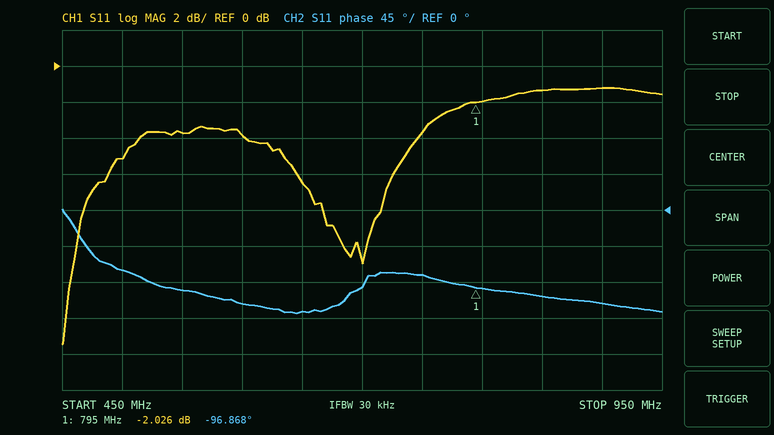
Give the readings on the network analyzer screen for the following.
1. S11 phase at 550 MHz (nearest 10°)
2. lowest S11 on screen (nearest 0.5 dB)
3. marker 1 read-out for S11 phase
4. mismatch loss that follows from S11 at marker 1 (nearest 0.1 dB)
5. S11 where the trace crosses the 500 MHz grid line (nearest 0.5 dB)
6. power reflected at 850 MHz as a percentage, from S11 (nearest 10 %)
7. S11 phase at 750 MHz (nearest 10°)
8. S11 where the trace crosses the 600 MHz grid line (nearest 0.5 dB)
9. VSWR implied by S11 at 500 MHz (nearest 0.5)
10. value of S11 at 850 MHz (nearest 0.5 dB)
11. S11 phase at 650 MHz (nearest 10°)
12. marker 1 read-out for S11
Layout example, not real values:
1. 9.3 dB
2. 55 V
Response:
1. -100°
2. -15.5 dB
3. -96.868°
4. 4.3 dB
5. -5.0 dB
6. 70 %
7. -80°
8. -4.0 dB
9. 3.5
10. -1.5 dB
11. -130°
12. -2.026 dB
